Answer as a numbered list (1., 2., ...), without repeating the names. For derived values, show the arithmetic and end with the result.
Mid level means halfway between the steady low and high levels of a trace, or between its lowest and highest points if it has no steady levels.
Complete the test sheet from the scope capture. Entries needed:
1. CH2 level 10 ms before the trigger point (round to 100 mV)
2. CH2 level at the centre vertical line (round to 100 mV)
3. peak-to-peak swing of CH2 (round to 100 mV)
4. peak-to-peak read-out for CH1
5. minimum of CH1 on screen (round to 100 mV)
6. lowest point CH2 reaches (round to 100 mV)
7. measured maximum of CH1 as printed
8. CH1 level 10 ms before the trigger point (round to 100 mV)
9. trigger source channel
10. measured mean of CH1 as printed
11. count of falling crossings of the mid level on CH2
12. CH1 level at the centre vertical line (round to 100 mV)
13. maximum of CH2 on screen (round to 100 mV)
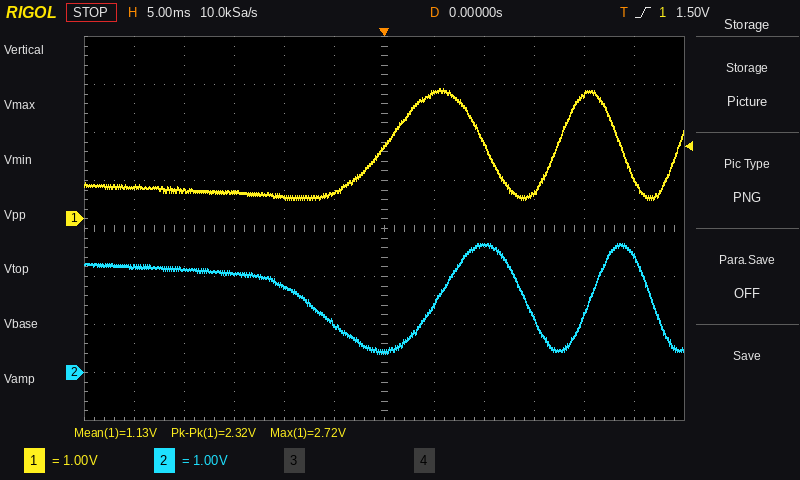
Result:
1. 1.8 V
2. 400 mV
3. 2.7 V − (400 mV) = 2.3 V
4. 2.32 V
5. 400 mV
6. 400 mV
7. 2.72 V
8. 400 mV
9. CH1
10. 1.13 V
11. 3
12. 1.5 V
13. 2.7 V
